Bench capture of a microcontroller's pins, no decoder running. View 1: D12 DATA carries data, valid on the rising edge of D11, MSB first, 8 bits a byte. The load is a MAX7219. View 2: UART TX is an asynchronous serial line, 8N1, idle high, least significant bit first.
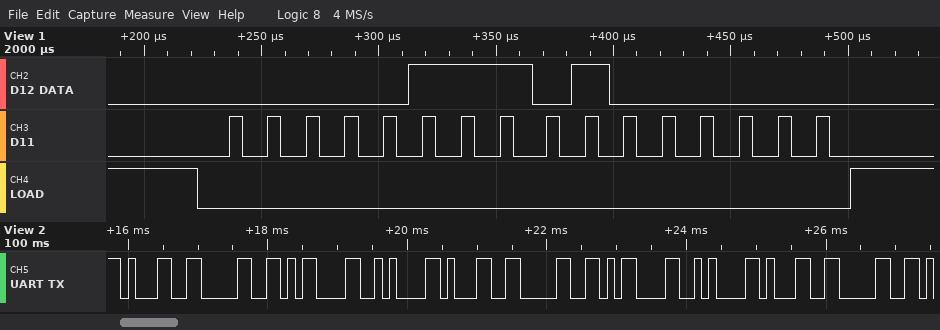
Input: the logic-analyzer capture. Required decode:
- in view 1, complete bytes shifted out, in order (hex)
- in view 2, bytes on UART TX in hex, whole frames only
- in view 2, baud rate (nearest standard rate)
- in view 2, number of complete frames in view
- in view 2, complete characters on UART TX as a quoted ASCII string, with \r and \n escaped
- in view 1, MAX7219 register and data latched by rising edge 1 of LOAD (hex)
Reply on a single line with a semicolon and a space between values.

07 40; 31 30 0D 0A 31 30 0D 0A 31 30; 9600 baud; 10; "10\r\n10\r\n10"; register 0x7, data 0x40
